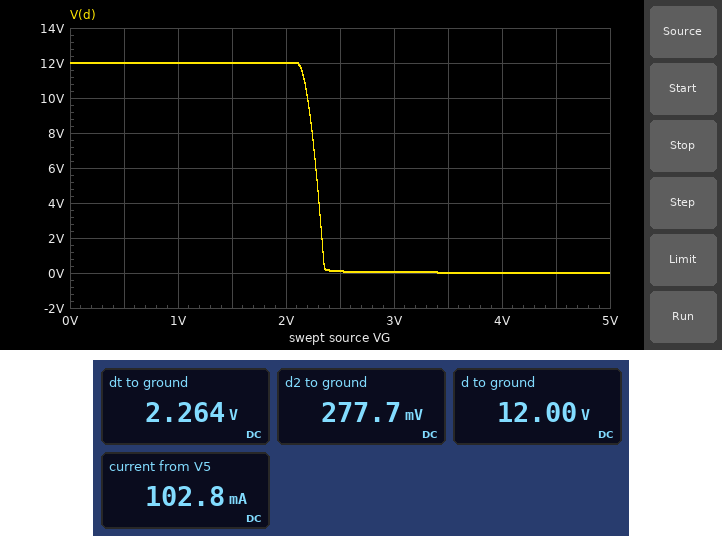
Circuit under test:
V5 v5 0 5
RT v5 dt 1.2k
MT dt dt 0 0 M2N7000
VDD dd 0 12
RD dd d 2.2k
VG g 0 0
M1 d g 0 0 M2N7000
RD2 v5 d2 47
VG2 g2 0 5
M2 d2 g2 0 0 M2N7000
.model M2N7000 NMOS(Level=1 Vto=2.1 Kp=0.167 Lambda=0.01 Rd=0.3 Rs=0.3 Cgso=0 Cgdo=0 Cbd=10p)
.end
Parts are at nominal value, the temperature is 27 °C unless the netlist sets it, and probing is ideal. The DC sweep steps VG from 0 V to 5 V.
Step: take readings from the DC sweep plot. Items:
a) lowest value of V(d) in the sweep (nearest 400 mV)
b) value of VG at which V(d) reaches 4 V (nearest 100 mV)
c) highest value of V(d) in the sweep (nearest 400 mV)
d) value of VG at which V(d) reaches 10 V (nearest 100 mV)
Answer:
0 V
2.3 V
12.0 V
2.2 V
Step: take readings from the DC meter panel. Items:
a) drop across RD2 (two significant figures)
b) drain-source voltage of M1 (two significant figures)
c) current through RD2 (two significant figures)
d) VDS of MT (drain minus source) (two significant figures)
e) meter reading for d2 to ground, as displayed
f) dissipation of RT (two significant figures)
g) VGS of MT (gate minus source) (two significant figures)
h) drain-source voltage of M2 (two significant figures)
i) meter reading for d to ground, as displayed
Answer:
4.7 V
12 V
100 mA
2.3 V
277.7 mV
6.2 mW
2.3 V
280 mV
12.00 V
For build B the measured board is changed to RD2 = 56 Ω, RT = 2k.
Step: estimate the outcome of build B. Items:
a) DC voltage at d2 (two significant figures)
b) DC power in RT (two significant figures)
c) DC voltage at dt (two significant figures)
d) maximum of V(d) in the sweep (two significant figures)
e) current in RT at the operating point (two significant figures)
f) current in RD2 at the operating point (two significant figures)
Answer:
230 mV
3.8 mW
2.2 V
12 V
1.4 mA
85 mA
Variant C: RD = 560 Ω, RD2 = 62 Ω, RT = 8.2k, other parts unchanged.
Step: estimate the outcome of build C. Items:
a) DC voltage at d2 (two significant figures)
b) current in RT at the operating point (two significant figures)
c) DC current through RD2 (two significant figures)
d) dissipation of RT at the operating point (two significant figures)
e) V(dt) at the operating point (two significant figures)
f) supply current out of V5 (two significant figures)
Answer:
210 mV
350 µA
77 mA
980 µW
2.2 V
78 mA
